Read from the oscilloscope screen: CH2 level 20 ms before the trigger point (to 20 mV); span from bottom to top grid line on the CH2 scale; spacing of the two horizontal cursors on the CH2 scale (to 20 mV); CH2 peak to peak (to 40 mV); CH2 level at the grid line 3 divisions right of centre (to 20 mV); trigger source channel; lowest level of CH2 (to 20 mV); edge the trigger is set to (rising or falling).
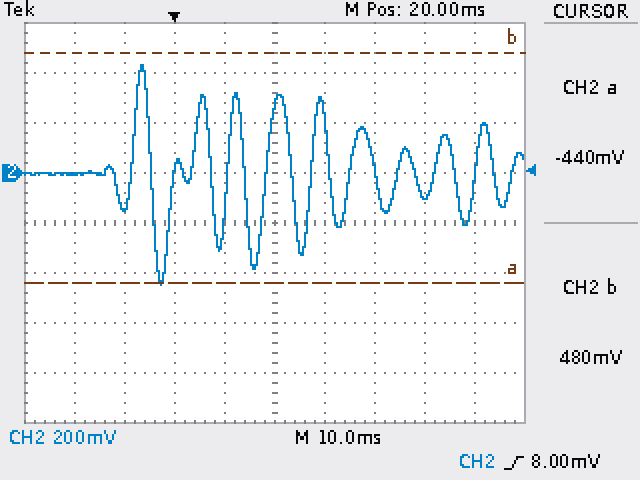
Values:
0 mV
1.6 V
920 mV
880 mV
-80 mV
CH2
-440 mV
rising
